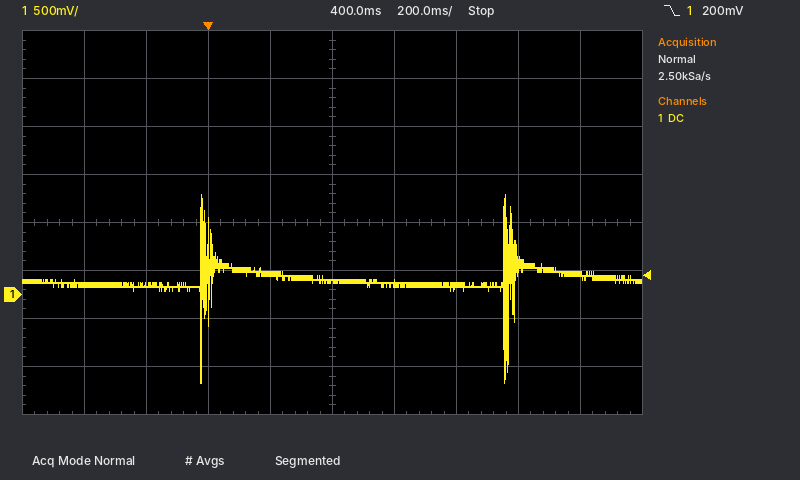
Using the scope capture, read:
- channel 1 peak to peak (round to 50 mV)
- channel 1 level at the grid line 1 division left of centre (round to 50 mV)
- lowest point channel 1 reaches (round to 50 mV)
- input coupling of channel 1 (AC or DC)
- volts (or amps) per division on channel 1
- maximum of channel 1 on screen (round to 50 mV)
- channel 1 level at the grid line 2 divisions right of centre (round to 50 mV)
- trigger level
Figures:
1.95 V
200 mV
-900 mV
DC
500 mV
1.05 V
100 mV
200 mV
